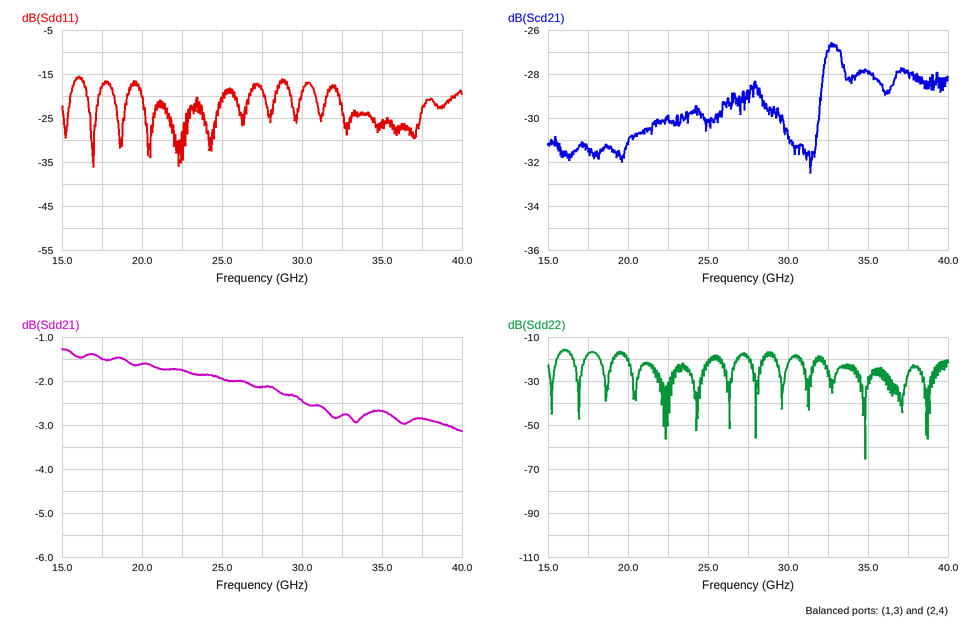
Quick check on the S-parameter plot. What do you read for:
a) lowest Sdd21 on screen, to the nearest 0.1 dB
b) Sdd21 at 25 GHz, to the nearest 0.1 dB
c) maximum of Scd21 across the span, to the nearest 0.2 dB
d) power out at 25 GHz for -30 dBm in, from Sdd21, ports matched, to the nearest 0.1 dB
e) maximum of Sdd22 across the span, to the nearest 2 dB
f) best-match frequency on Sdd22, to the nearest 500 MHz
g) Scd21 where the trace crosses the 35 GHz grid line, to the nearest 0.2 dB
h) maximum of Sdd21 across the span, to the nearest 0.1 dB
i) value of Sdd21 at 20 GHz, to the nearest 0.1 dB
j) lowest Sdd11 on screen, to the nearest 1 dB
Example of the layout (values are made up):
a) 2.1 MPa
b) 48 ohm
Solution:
a) -3.1 dB
b) -1.9 dB
c) -26.6 dB
d) -31.9 dBm
e) -16 dB
f) 35.0 GHz
g) -28.0 dB
h) -1.3 dB
i) -1.6 dB
j) -36 dB
